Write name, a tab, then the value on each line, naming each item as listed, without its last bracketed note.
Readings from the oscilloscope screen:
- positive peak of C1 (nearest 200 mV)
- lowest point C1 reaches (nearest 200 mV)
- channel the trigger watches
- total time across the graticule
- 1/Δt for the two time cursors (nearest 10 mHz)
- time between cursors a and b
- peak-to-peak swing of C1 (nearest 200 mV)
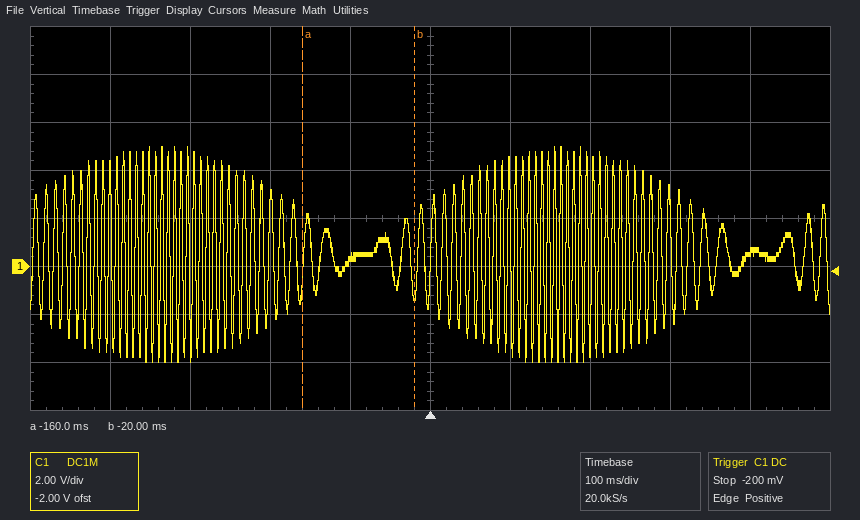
positive peak of C1	5.0 V
lowest point C1 reaches	-4.0 V
channel the trigger watches	C1
total time across the graticule	1 s
1/Δt for the two time cursors	7.14 Hz
time between cursors a and b	140 ms
peak-to-peak swing of C1	9.0 V
